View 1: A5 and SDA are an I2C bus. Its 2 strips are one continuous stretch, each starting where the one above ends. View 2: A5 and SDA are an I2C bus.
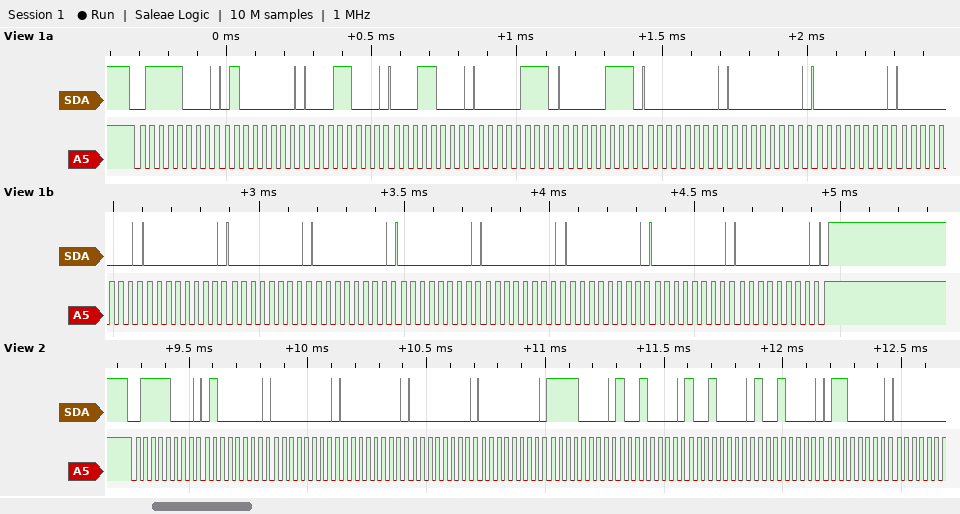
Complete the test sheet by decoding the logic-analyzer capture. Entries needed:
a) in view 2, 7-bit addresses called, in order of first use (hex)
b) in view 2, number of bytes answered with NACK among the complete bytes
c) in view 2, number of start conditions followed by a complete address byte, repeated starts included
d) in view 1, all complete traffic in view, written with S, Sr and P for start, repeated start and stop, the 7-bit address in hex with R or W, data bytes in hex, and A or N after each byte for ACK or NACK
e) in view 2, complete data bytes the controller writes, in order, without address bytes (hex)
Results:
0x3C
0
1
S 3CW A 40 A 18 A 18 A 07 A 07 A 00 A 00 A 00 A 00 A 00 A 00 A 00 A 00 A 00 A 00 A 00 A 00 A P
40 00 00 00 00 F0 90 90 90 60
